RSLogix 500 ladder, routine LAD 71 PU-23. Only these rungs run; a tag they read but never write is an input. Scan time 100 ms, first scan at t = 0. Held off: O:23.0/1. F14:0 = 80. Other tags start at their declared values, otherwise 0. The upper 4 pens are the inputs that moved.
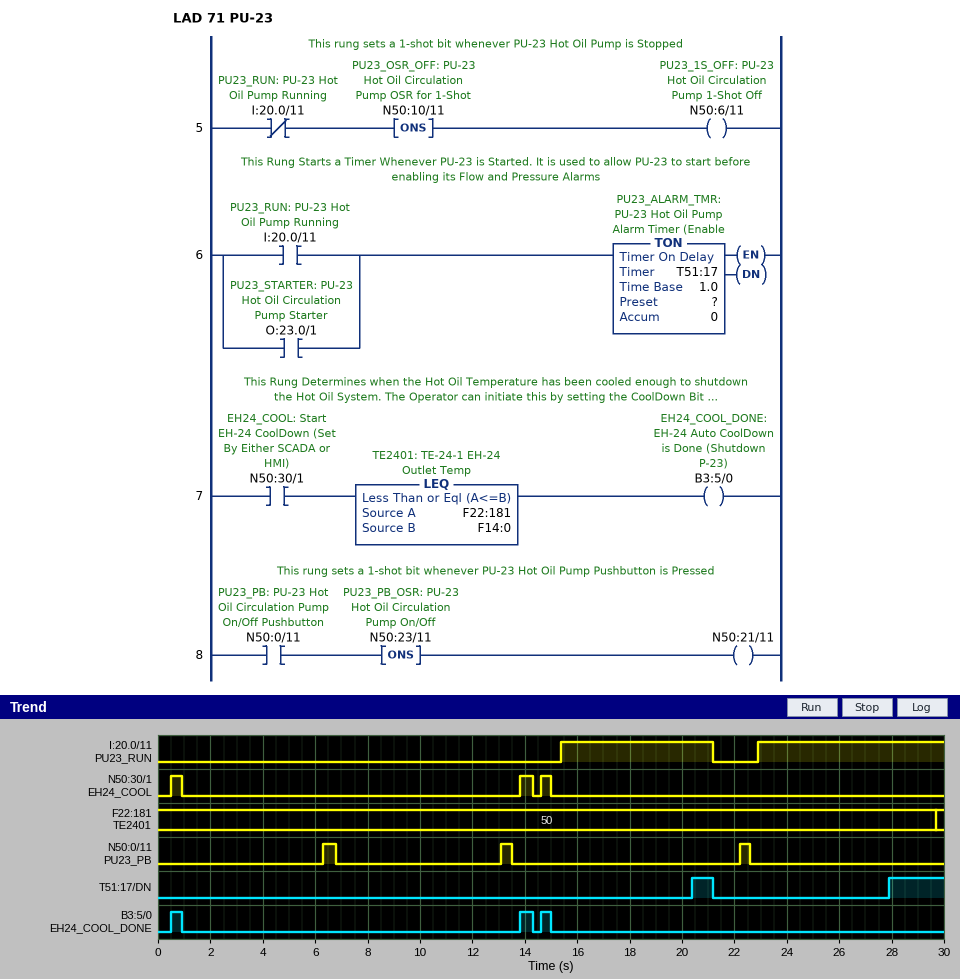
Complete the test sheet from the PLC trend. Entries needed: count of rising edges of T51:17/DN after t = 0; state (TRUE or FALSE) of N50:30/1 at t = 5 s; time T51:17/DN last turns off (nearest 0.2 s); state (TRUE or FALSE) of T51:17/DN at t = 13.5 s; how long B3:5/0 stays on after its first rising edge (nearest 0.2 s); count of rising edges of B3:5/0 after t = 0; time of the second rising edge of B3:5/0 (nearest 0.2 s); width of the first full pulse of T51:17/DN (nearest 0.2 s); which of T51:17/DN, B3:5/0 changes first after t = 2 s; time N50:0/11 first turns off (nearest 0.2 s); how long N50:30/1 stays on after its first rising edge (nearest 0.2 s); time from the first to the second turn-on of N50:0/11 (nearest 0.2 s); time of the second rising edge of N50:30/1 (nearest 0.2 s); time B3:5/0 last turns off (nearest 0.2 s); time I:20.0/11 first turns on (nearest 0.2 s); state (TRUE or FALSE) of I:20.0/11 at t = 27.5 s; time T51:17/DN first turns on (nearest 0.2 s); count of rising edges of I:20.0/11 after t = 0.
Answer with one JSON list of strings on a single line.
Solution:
["2", "FALSE", "21.2 s", "FALSE", "0.4 s", "3", "13.8 s", "0.8 s", "B3:5/0", "6.8 s", "0.4 s", "6.8 s", "13.8 s", "15.0 s", "15.4 s", "TRUE", "20.4 s", "2"]
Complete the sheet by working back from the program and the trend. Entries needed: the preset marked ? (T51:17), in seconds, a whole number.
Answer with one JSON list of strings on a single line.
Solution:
["5 s"]
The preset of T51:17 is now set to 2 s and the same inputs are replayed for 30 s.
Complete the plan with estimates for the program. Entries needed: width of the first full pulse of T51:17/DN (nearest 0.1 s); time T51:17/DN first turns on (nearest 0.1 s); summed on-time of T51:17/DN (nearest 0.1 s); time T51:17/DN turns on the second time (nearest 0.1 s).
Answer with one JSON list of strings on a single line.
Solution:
["3.8 s", "17.4 s", "8.9 s", "24.9 s"]
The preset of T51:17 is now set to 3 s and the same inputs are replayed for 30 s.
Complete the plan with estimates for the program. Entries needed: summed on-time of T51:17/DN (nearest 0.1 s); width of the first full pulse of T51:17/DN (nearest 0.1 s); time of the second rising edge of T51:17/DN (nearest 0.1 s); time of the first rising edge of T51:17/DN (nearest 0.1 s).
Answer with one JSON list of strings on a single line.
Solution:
["6.9 s", "2.8 s", "25.9 s", "18.4 s"]
